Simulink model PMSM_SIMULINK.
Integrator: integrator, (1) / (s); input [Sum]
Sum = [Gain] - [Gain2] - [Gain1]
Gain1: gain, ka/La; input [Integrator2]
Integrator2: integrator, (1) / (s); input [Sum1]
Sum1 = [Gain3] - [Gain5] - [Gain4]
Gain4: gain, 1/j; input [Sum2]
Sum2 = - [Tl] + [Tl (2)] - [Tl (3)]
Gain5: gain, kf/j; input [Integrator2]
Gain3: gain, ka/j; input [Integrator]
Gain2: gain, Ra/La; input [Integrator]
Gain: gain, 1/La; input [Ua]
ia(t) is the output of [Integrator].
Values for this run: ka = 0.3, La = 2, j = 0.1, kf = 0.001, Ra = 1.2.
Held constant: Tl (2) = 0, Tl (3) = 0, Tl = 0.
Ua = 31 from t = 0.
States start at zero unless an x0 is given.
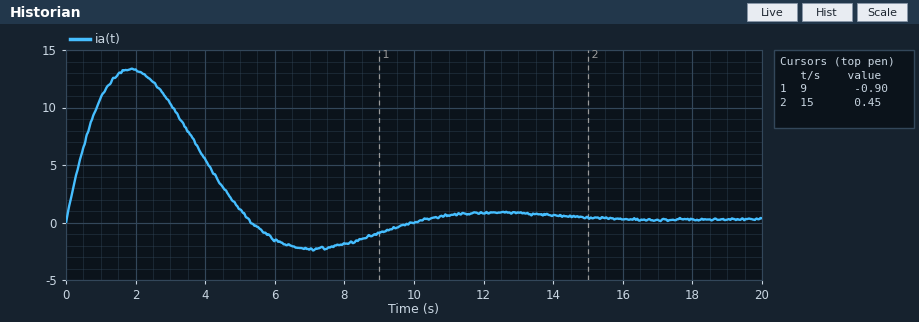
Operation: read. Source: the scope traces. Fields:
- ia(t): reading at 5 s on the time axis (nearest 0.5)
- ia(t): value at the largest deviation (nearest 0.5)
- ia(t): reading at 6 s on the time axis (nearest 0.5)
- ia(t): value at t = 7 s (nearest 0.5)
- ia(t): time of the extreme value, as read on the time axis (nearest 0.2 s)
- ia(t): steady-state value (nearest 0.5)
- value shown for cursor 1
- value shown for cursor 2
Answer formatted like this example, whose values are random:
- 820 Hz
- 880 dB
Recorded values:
- 1.0
- 13.5
- -1.5
- -2.5
- 1.8 s
- 0.5
- -0.90
- 0.45
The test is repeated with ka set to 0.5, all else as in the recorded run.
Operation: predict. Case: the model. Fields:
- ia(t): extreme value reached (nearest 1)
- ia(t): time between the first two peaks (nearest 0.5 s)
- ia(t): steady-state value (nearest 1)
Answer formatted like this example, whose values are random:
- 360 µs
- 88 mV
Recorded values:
- 10
- 6.0 s
- 0
